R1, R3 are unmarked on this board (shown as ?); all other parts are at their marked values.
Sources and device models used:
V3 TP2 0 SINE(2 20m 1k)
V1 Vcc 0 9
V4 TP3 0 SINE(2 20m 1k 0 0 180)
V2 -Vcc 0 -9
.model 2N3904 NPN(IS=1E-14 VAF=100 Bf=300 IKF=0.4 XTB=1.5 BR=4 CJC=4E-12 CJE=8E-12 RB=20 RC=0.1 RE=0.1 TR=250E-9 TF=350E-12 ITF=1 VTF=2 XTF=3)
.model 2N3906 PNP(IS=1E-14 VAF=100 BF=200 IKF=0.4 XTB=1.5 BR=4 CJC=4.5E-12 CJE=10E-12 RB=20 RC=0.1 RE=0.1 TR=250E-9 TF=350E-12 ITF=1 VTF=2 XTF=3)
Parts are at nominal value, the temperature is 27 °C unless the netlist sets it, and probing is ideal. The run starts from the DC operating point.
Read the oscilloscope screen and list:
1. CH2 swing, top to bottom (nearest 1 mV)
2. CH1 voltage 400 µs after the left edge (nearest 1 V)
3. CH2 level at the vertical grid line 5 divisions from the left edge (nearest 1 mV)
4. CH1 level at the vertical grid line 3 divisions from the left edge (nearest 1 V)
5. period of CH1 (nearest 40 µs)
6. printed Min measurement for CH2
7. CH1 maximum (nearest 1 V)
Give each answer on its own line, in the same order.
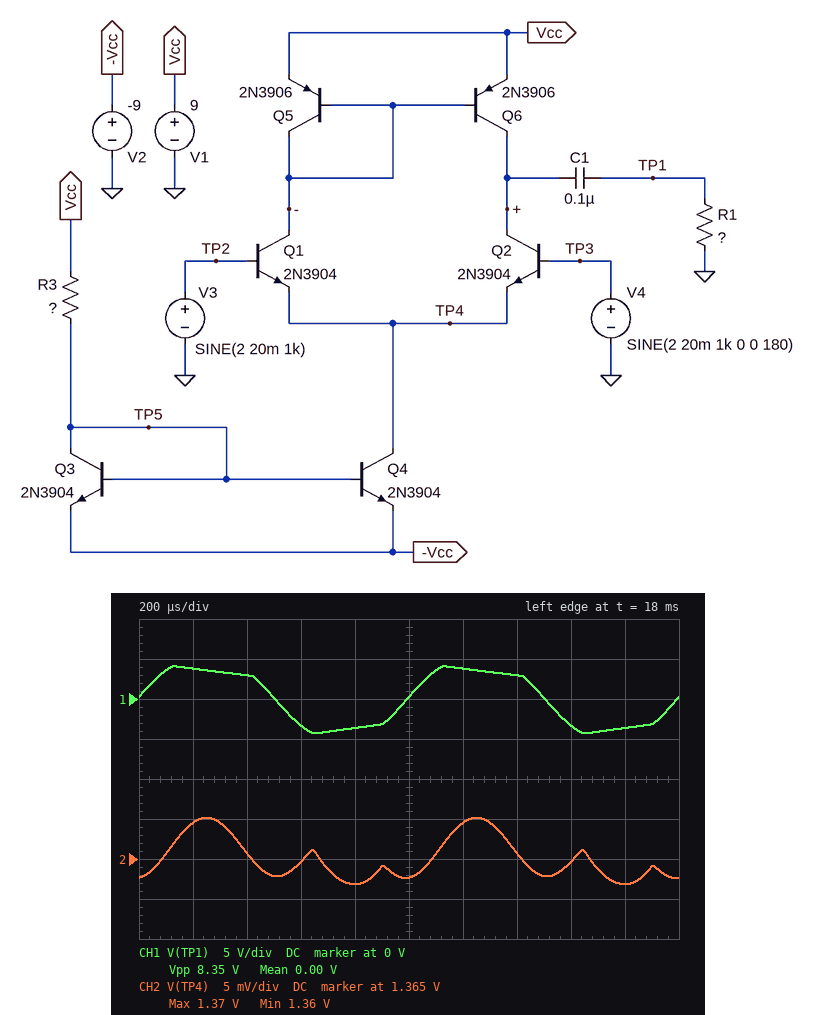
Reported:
8 mV
3 V
1.363 V
-3 V
1.00 ms
1.36 V
4 V
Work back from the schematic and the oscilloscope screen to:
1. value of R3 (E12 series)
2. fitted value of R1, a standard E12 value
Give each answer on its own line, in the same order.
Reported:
18 kΩ
8.2 kΩ
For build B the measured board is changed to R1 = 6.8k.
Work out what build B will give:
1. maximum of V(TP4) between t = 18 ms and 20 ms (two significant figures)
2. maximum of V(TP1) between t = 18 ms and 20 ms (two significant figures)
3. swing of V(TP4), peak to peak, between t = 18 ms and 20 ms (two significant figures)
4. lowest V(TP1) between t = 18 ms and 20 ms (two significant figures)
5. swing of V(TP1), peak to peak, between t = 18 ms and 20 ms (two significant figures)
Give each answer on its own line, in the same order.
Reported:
1.4 V
3.9 V
7.5 mV
-4.1 V
8.1 V
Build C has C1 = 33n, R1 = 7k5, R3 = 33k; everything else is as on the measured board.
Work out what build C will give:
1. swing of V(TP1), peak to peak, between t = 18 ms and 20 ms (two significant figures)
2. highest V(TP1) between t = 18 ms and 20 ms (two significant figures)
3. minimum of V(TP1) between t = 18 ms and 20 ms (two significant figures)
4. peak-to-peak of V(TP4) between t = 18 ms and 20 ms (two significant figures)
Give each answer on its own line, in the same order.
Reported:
5.4 V
2.7 V
-2.7 V
7.6 mV
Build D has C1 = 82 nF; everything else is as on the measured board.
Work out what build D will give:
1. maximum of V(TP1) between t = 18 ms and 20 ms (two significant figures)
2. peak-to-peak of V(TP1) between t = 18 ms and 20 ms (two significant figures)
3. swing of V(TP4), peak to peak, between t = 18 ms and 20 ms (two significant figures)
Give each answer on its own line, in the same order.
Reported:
4.2 V
8.5 V
8.6 mV
